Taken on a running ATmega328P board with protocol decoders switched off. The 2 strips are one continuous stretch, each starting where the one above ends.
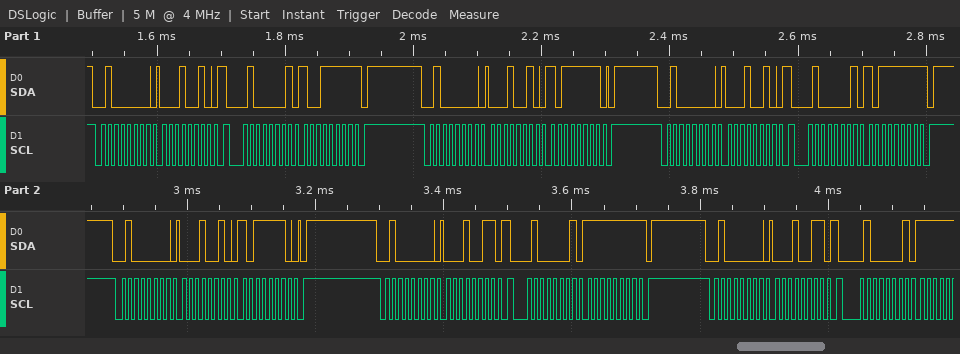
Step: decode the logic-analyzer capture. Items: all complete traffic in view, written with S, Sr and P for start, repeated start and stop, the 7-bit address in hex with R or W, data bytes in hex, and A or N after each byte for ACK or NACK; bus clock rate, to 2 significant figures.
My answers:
S 20W A 12 A Sr 20R A 9F N P S 20W A 12 A BF A P S 20W A 12 A Sr 20R A BF N P S 20W A 12 A BE A P S 20W A 13 A Sr 20R A FF N P S 20W A 13 A Sr 20R A
100 kHz
